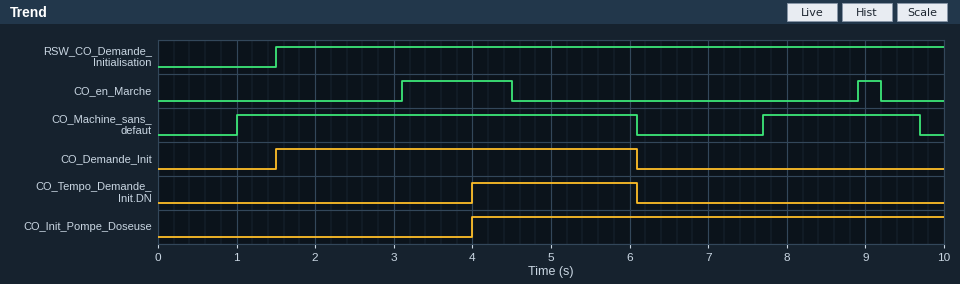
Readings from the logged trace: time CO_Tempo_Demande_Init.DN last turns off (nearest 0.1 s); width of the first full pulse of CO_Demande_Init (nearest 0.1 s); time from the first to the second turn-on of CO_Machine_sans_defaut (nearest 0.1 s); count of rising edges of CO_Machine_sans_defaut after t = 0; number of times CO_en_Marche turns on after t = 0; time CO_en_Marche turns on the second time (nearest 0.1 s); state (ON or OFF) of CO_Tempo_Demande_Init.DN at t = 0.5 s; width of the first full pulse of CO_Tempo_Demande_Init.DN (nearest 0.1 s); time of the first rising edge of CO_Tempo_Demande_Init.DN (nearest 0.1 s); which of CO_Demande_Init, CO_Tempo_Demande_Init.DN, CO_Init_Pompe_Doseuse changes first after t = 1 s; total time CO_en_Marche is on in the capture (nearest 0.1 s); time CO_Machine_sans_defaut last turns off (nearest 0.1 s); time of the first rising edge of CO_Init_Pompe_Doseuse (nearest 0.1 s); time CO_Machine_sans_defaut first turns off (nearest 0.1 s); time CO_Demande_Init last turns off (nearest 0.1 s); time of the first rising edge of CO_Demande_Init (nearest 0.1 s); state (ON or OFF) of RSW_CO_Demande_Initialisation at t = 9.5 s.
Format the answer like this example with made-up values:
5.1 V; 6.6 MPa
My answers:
6.1 s; 4.6 s; 6.7 s; 2; 2; 8.9 s; OFF; 2.1 s; 4.0 s; CO_Demande_Init; 1.7 s; 9.7 s; 4.0 s; 6.1 s; 6.1 s; 1.5 s; ON
